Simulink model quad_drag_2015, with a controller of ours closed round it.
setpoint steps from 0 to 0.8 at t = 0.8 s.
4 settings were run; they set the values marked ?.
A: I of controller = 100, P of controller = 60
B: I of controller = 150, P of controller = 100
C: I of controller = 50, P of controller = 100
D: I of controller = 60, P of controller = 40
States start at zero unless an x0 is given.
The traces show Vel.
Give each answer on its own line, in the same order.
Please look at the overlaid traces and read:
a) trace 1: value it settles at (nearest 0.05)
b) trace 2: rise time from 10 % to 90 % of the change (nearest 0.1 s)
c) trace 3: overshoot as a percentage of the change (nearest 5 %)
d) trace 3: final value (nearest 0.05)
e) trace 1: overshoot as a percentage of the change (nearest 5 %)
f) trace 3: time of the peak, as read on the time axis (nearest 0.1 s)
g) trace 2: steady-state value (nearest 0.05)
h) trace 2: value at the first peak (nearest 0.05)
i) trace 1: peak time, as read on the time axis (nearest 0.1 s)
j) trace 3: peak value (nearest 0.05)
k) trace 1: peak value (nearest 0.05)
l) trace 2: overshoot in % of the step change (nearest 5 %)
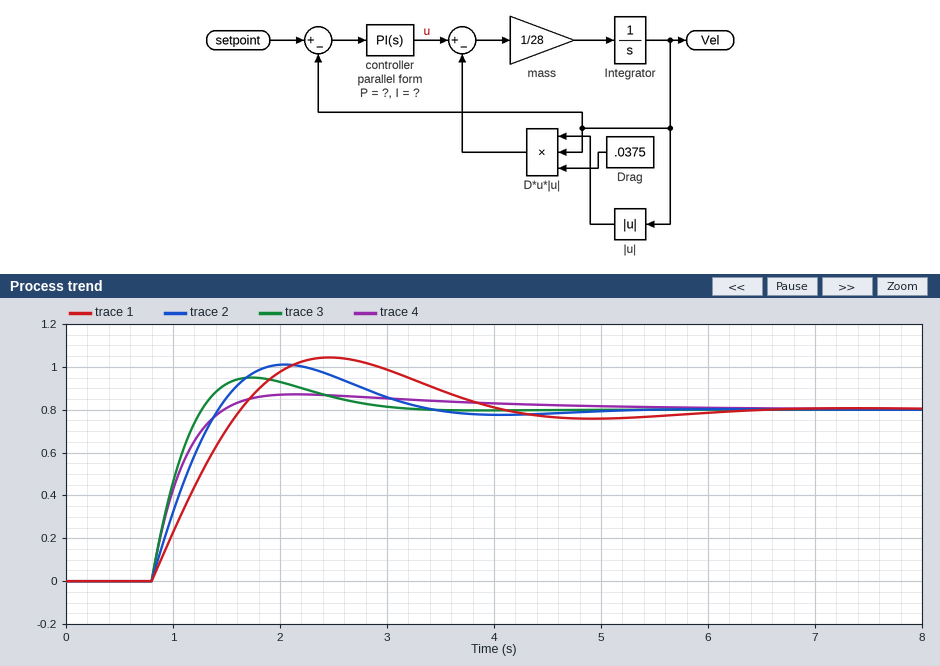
0.80
0.5 s
20 %
0.80
30 %
1.7 s
0.80
1.00
2.5 s
0.95
1.05
25 %
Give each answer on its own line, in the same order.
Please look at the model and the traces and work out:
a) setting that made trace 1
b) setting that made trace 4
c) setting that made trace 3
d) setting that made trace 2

D
C
B
A
